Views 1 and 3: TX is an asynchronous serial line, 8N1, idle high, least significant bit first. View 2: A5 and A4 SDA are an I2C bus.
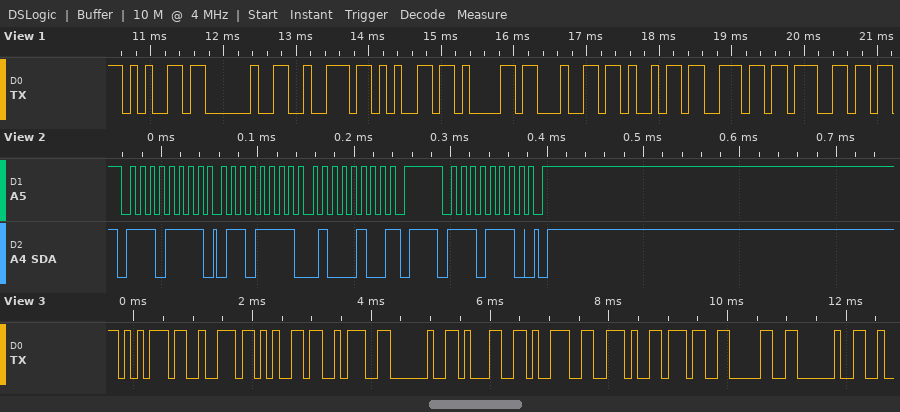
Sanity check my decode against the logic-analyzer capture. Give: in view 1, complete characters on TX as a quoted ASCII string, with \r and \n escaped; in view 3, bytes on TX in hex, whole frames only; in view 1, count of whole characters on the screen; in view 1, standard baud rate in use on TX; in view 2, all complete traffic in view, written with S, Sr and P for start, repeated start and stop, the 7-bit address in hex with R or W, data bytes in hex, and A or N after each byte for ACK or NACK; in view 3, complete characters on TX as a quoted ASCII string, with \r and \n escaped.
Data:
"e reading"
0x75 0x72 0x65 0x3A 0x20 0x31 0x39 0x2E 0x37 0x30 0x20
9
9600 baud
S 77R A 6F A 44 N P S 77W A P
"ure: 19.70 "
